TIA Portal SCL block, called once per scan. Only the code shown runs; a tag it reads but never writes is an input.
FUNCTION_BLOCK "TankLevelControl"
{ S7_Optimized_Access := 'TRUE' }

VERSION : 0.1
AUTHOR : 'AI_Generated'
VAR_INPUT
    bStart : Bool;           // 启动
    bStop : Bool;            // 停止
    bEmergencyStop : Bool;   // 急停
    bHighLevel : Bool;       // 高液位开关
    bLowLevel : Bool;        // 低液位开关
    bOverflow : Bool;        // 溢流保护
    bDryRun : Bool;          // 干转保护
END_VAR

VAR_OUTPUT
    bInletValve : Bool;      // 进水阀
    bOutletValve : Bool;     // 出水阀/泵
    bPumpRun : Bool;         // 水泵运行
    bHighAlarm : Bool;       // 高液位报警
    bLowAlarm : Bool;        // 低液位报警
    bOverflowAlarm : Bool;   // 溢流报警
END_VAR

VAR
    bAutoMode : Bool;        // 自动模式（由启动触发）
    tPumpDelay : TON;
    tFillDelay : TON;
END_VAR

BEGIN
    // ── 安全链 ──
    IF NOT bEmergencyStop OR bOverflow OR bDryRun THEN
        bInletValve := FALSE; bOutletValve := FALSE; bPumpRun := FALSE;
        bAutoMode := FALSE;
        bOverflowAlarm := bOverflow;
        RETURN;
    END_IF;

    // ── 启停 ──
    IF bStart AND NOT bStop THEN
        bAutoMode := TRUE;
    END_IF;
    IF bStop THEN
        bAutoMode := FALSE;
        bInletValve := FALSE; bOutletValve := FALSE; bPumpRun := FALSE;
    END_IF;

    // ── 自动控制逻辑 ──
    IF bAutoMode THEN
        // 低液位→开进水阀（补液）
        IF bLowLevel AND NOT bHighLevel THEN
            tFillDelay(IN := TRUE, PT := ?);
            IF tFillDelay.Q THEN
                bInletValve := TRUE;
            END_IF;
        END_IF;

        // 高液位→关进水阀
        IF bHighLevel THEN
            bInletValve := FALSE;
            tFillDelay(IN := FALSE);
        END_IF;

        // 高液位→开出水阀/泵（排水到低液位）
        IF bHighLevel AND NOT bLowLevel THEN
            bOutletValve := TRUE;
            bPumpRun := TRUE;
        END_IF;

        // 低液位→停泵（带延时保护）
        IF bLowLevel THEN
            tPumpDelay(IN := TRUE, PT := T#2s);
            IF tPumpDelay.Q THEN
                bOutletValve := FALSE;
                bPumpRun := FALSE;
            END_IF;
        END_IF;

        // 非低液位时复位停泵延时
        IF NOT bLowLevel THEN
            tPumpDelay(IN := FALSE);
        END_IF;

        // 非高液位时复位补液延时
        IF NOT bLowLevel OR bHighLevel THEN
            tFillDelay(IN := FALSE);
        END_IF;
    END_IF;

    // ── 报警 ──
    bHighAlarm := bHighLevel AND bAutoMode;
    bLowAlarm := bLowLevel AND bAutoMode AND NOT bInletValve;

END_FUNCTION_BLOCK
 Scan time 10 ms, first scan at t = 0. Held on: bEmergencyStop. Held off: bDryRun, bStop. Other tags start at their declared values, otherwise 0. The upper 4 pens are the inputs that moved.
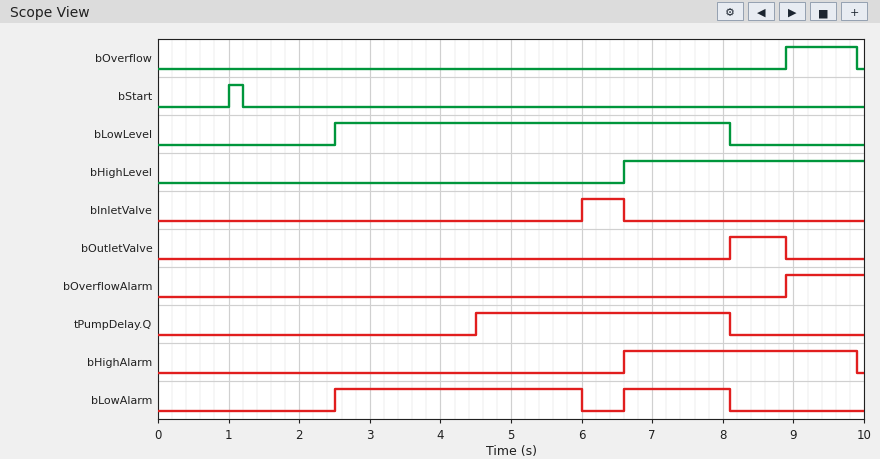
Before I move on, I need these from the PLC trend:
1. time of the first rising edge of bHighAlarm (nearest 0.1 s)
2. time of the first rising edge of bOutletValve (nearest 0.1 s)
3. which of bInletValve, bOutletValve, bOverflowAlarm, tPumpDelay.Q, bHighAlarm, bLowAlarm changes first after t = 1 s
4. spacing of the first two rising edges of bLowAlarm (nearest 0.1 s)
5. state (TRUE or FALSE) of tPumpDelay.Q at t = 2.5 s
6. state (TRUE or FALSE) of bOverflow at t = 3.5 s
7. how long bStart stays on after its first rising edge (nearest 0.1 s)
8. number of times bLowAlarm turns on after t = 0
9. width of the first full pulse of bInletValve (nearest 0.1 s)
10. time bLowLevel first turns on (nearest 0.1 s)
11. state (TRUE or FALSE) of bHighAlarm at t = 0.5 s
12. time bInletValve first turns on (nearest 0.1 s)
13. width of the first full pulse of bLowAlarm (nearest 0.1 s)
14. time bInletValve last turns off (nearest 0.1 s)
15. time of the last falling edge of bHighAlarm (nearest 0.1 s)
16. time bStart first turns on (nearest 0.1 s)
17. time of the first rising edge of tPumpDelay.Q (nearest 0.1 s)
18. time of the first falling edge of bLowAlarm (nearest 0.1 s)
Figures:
6.6 s
8.1 s
bLowAlarm
4.1 s
FALSE
FALSE
0.2 s
2
0.6 s
2.5 s
FALSE
6.0 s
3.5 s
6.6 s
9.9 s
1.0 s
4.5 s
6.0 s
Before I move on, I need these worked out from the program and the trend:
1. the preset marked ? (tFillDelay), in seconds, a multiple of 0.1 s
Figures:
3.5 s
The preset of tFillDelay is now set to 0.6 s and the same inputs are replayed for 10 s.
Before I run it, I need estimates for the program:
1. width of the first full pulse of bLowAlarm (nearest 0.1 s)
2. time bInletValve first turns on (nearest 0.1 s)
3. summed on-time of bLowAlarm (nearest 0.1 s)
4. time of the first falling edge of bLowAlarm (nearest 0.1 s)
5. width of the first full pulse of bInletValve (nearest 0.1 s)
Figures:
0.6 s
3.1 s
2.1 s
3.1 s
3.5 s
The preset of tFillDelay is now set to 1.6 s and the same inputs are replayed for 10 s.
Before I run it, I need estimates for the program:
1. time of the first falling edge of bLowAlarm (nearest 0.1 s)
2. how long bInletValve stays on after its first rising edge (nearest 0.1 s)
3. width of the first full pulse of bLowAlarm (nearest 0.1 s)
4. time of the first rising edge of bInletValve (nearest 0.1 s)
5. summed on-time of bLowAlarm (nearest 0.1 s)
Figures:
4.1 s
2.5 s
1.6 s
4.1 s
3.1 s
